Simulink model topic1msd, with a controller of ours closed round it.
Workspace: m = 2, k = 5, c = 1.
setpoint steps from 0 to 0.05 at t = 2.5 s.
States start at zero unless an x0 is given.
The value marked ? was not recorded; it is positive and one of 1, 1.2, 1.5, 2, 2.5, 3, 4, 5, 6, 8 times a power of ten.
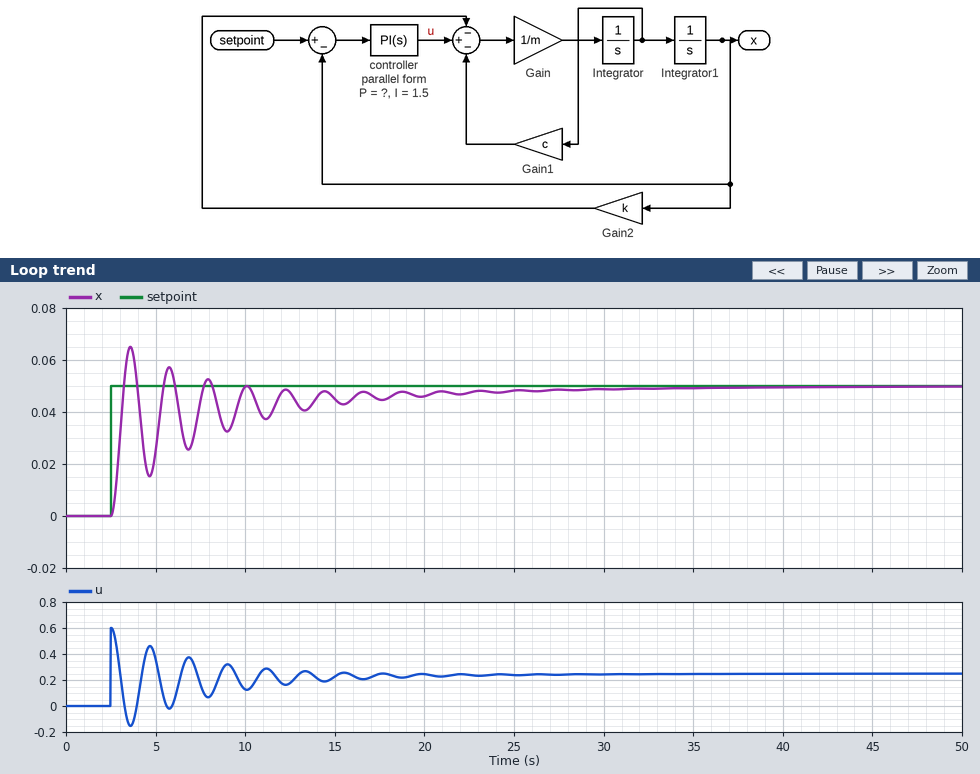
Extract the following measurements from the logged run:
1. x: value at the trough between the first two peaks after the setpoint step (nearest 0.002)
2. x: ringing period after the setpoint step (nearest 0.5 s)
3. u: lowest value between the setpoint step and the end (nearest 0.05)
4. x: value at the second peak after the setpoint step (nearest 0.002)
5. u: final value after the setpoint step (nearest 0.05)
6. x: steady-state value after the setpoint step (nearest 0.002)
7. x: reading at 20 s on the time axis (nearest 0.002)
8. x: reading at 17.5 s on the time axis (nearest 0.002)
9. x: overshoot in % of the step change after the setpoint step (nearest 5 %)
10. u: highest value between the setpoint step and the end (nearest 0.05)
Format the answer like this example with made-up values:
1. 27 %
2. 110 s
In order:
1. 0.016
2. 2.0 s
3. -0.15
4. 0.058
5. 0.25
6. 0.050
7. 0.046
8. 0.044
9. 30 %
10. 0.60
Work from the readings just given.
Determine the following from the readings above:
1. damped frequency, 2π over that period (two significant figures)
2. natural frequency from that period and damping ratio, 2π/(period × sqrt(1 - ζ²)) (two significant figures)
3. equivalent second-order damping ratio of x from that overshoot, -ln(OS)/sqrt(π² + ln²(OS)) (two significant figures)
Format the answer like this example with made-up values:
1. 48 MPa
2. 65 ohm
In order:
1. 3.1 rad/s
2. 3.4 rad/s
3. 0.36
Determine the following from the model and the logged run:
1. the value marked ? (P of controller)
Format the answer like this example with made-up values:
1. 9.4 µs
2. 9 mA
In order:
1. 12
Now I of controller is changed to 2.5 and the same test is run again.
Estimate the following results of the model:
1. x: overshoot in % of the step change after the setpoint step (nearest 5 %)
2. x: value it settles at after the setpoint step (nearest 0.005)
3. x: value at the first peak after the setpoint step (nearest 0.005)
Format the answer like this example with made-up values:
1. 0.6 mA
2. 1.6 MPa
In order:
1. 35 %
2. 0.050
3. 0.065
